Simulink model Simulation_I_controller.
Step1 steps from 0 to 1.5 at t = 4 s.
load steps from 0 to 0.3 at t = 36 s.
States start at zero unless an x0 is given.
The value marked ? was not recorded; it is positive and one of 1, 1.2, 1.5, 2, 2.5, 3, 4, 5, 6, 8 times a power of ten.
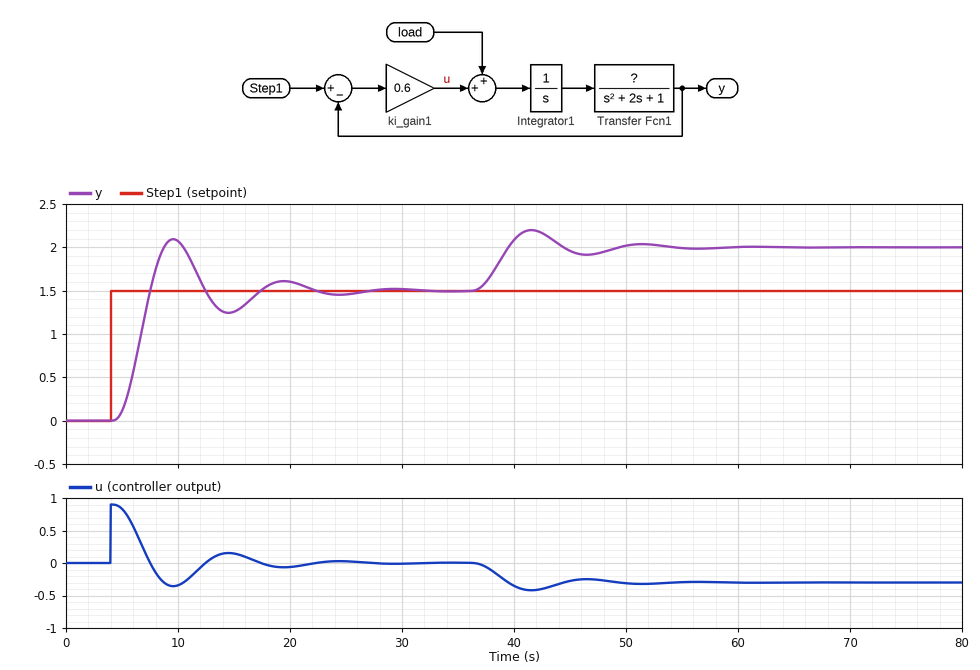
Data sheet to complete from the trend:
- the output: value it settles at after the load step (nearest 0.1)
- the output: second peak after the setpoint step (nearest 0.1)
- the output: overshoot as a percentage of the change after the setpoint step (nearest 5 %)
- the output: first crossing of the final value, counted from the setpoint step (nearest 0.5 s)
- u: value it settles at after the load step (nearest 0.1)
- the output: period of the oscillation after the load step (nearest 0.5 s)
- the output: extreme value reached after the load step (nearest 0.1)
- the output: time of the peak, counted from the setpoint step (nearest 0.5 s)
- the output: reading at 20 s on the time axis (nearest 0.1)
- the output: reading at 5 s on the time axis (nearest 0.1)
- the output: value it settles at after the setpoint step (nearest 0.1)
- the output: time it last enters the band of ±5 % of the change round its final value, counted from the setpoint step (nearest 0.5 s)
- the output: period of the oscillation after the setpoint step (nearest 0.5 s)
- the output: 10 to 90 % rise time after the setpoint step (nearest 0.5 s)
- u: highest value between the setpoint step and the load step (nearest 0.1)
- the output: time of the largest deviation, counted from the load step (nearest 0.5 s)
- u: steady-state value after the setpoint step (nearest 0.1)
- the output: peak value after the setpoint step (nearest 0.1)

2.0
1.6
40 %
3.5 s
-0.3
10.0 s
2.2
5.5 s
1.6
0.1
1.5
17.0 s
10.0 s
2.0 s
0.9
5.5 s
0.0
2.1
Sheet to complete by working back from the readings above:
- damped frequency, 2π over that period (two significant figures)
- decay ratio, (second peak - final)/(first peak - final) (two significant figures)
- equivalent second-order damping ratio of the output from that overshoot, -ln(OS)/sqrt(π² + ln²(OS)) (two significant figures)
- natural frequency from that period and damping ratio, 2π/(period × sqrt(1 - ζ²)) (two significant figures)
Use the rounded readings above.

0.63 rad/s
0.17
0.28
0.65 rad/s
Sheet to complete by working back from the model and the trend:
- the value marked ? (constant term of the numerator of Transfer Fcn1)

1.2
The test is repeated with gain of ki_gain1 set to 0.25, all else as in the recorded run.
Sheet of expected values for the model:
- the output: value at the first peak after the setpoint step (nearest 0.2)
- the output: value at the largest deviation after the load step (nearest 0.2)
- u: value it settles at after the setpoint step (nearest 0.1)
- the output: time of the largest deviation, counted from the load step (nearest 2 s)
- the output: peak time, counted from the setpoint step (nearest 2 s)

1.6
2.8
0.0
10 s
10 s
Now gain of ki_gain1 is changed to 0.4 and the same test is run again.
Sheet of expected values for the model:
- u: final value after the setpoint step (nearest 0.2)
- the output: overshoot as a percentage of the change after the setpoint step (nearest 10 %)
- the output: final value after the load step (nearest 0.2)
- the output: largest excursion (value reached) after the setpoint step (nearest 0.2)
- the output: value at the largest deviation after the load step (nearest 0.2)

0.0
20 %
2.2
1.8
2.4
